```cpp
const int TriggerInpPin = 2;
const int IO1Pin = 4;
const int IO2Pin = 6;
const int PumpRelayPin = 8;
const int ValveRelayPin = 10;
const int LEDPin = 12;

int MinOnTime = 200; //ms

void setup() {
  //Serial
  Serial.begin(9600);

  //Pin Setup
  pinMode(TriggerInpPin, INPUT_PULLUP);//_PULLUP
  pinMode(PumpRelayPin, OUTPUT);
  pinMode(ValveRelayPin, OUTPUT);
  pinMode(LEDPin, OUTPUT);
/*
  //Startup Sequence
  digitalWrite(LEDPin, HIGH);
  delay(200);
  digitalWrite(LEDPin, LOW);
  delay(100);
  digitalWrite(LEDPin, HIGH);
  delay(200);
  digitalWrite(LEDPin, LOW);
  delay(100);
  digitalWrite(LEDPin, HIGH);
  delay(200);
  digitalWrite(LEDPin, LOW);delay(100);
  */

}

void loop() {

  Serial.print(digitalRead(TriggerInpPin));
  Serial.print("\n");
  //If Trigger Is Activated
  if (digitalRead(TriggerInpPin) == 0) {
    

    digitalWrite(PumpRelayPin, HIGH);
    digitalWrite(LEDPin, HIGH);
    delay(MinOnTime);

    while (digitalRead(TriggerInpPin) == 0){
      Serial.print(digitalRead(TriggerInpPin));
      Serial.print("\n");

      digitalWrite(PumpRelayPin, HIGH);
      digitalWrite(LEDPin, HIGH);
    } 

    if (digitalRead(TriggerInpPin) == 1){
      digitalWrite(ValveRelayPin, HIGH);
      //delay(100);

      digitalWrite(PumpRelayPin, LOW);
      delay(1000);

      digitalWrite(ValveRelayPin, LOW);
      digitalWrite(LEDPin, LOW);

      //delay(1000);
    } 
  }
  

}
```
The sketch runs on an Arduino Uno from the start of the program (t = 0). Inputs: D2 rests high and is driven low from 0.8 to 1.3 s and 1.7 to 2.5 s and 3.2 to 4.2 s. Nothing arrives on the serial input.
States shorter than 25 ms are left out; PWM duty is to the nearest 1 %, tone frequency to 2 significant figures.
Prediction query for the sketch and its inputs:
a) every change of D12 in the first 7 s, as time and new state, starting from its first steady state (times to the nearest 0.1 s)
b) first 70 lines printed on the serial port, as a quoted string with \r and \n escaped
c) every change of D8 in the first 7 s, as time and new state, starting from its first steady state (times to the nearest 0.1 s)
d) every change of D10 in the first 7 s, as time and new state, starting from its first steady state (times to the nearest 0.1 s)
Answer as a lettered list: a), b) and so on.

a) 0 s low; 0.8 s high; 5.2 s low
b) "1\n1\n1\n1\n1\n1\n1\n1\n1\n1\n1\n1\n1\n1\n1\n1\n1\n1\n1\n1\n1\n1\n1\n1\n1\n1\n1\n1\n1\n1\n1\n1\n1\n1\n1\n1\n1\n1\n1\n1\n1\n1\n1\n1\n1\n1\n1\n1\n1\n1\n1\n1\n1\n1\n1\n1\n1\n1\n1\n1\n1\n1\n1\n1\n1\n1\n1\n1\n1\n1\n"
c) 0 s low; 0.8 s high; 1.3 s low; 2.3 s high; 2.5 s low; 3.5 s high; 4.2 s low
d) 0 s low; 1.3 s high; 2.3 s low; 2.5 s high; 3.5 s low; 4.2 s high; 5.2 s low
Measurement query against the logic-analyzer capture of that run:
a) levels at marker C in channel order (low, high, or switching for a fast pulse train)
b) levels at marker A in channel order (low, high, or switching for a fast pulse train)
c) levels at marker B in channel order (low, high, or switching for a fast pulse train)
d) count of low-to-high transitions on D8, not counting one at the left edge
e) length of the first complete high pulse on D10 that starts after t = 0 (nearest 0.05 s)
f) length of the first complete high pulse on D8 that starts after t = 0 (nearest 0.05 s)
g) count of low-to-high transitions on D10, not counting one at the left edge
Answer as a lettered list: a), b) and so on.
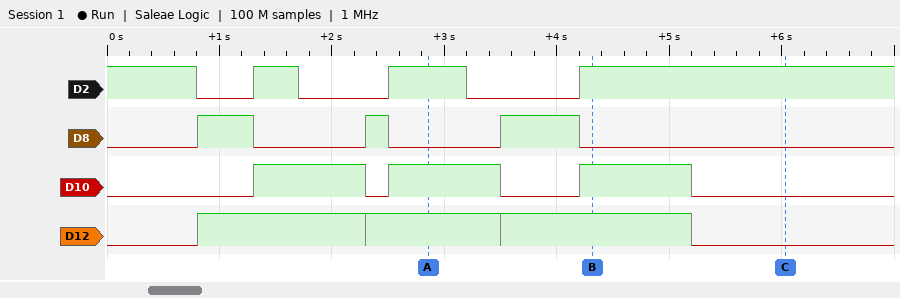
a) D2 high, D8 low, D10 low, D12 low
b) D2 high, D8 low, D10 high, D12 high
c) D2 high, D8 low, D10 high, D12 high
d) 3
e) 1.00 s
f) 0.50 s
g) 3
